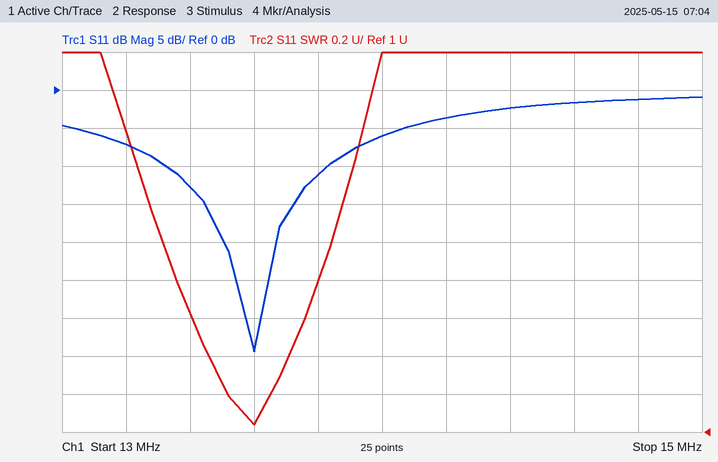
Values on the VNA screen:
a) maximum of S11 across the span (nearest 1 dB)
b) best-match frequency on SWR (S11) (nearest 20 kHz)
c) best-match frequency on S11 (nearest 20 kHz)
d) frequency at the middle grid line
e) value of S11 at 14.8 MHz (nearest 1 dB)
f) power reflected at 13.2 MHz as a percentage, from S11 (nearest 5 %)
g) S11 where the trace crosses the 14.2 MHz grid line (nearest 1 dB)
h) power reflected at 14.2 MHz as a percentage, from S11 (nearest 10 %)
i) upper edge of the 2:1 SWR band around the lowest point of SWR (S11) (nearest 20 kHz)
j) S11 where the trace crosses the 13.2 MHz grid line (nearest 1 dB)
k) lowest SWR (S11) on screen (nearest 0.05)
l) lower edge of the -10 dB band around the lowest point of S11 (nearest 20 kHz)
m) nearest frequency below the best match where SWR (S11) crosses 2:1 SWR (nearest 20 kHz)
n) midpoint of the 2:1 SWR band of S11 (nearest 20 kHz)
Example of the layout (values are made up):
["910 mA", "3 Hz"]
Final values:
["-1 dB", "13.60 MHz", "13.60 MHz", "14 MHz", "-1 dB", "20 %", "-4 dB", "40 %", "13.84 MHz", "-7 dB", "1.05", "13.32 MHz", "13.32 MHz", "13.58 MHz"]
